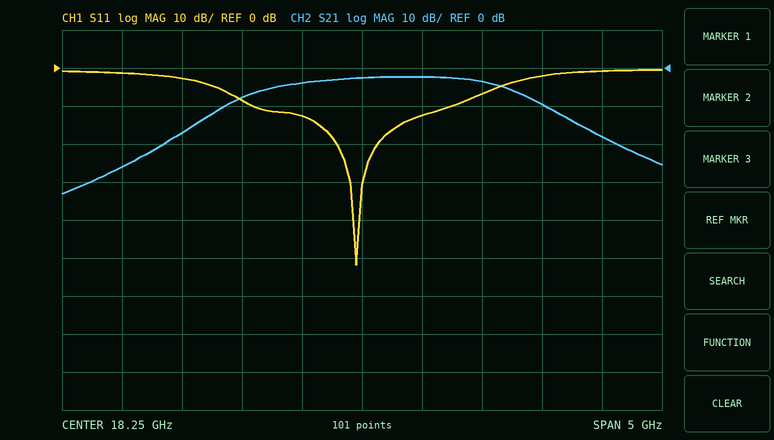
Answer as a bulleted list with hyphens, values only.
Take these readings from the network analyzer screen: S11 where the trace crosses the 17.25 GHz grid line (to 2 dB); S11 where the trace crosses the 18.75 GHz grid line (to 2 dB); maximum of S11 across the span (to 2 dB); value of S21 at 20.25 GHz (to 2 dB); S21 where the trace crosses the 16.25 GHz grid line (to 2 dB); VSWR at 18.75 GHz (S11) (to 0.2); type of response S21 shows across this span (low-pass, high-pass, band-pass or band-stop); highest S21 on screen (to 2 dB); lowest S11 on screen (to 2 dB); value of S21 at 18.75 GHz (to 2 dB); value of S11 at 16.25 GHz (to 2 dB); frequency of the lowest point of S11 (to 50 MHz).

- -8 dB
- -12 dB
- 0 dB
- -18 dB
- -26 dB
- 1.6
- band-pass
- -2 dB
- -52 dB
- -2 dB
- -2 dB
- 18.20 GHz
